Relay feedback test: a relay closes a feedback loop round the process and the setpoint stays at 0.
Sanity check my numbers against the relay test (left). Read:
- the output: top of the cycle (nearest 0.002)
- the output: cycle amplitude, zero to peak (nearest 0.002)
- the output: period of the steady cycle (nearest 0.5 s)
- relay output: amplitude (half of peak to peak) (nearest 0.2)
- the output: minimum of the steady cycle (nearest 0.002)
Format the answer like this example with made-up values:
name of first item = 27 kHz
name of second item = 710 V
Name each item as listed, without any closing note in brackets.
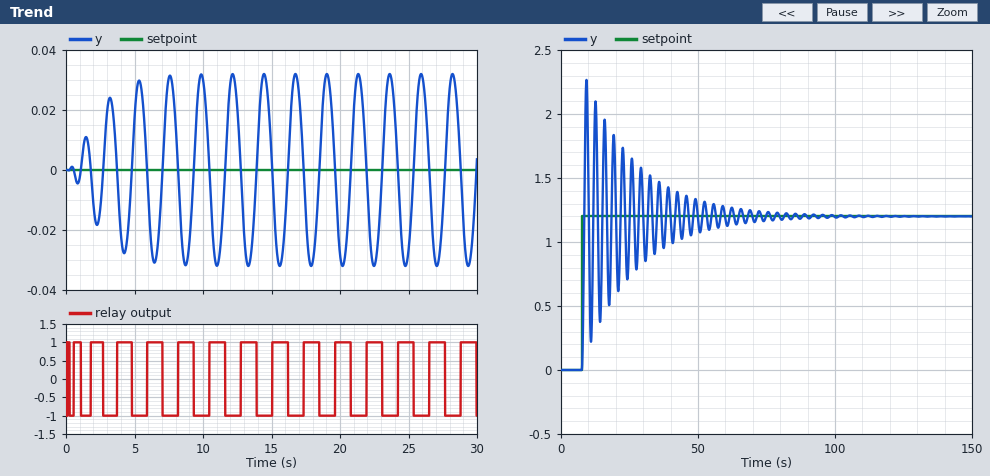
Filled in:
the output: top of the cycle = 0.032
the output: cycle amplitude, zero to peak = 0.032
the output: period of the steady cycle = 2.5 s
relay output: amplitude (half of peak to peak) = 1.0
the output: minimum of the steady cycle = -0.032
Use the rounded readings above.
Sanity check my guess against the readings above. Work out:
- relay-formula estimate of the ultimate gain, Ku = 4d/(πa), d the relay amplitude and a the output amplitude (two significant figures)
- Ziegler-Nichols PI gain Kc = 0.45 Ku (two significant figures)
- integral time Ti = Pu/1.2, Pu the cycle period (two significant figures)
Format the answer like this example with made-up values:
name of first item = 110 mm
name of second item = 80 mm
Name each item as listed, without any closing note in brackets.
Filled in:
relay-formula estimate of the ultimate gain, Ku = 4d/(πa), d the relay amplitude and a the output amplitude = 40
Ziegler-Nichols PI gain Kc = 0.45 Ku = 18
integral time Ti = Pu/1.2, Pu the cycle period = 2.1 s
